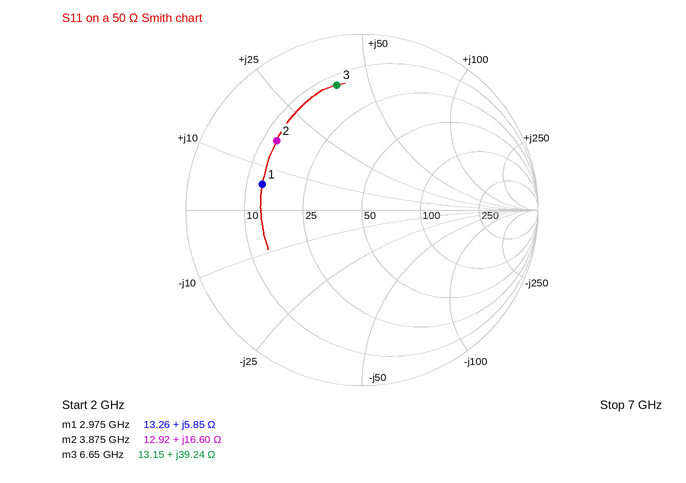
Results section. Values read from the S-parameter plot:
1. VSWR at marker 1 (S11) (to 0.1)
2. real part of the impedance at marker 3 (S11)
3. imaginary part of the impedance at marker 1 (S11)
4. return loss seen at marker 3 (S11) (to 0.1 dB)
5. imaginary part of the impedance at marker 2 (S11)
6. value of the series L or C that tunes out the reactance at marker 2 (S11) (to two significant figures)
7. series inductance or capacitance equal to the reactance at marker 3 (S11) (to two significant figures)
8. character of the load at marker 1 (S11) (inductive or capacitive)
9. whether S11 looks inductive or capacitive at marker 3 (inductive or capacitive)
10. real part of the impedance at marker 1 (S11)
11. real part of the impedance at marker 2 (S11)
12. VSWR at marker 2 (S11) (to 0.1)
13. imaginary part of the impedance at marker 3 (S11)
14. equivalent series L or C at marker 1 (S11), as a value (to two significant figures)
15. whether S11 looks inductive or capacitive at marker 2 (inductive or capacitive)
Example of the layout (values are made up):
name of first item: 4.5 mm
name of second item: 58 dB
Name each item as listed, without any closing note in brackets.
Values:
VSWR at marker 1 (S11): 3.8
real part of the impedance at marker 3: 13.15 Ω
imaginary part of the impedance at marker 1: +5.85 Ω
return loss seen at marker 3 (S11): 2.8 dB
imaginary part of the impedance at marker 2: +16.60 Ω
value of the series L or C that tunes out the reactance at marker 2 (S11): 2.5 pF
series inductance or capacitance equal to the reactance at marker 3 (S11): 940 pH
character of the load at marker 1 (S11): inductive
whether S11 looks inductive or capacitive at marker 3: inductive
real part of the impedance at marker 1: 13.26 Ω
real part of the impedance at marker 2: 12.92 Ω
VSWR at marker 2 (S11): 4.3
imaginary part of the impedance at marker 3: +39.24 Ω
equivalent series L or C at marker 1 (S11), as a value: 310 pH
whether S11 looks inductive or capacitive at marker 2: inductive
